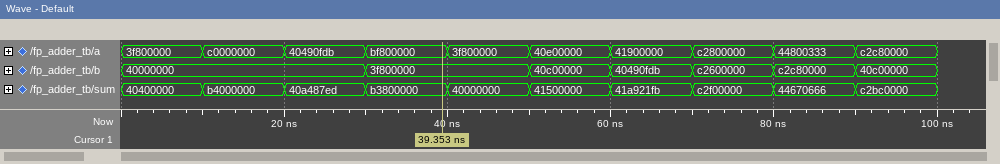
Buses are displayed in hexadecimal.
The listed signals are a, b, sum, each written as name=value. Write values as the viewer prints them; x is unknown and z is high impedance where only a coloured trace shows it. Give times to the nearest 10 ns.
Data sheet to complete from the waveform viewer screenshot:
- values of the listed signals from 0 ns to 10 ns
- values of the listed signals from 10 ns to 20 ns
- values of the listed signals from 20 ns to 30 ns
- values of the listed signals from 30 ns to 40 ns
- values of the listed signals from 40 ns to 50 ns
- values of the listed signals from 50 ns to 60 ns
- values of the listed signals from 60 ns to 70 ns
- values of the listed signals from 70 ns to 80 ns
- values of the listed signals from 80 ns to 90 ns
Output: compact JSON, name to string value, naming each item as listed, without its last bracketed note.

{"values of the listed signals from 0 ns to 10 ns": "a=3f800000, b=40000000, sum=40400000", "values of the listed signals from 10 ns to 20 ns": "a=c0000000, b=40000000, sum=b4000000", "values of the listed signals from 20 ns to 30 ns": "a=40490fdb, b=40000000, sum=40a487ed", "values of the listed signals from 30 ns to 40 ns": "a=bf800000, b=3f800000, sum=b3800000", "values of the listed signals from 40 ns to 50 ns": "a=3f800000, b=3f800000, sum=40000000", "values of the listed signals from 50 ns to 60 ns": "a=40e00000, b=40c00000, sum=41500000", "values of the listed signals from 60 ns to 70 ns": "a=41900000, b=40490fdb, sum=41a921fb", "values of the listed signals from 70 ns to 80 ns": "a=c2800000, b=c2600000, sum=c2f00000", "values of the listed signals from 80 ns to 90 ns": "a=44800333, b=c2c80000, sum=44670666"}
